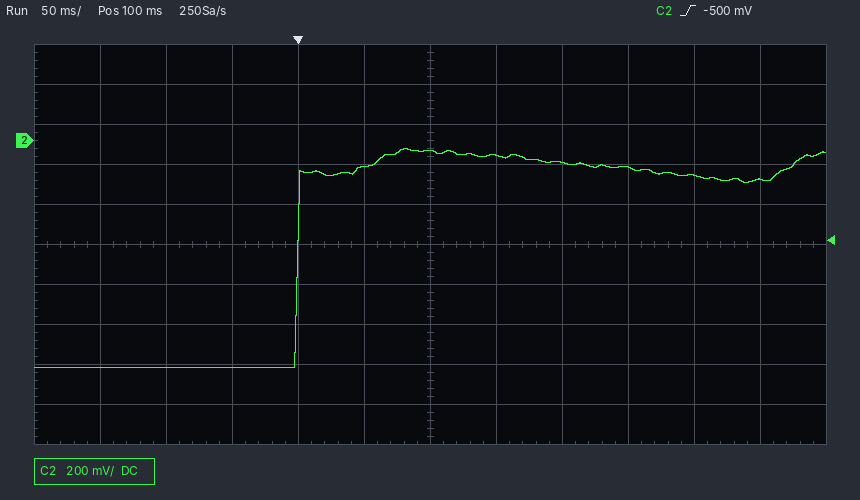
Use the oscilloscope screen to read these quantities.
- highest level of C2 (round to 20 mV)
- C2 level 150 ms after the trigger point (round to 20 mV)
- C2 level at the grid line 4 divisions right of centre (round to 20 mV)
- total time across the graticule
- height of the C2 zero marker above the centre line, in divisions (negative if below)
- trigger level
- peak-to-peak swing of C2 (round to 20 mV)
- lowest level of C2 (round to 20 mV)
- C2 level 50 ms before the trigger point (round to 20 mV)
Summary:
-40 mV
-80 mV
-180 mV
600 ms
+2.6 div
-500 mV
1.10 V
-1.14 V
-1.14 V
